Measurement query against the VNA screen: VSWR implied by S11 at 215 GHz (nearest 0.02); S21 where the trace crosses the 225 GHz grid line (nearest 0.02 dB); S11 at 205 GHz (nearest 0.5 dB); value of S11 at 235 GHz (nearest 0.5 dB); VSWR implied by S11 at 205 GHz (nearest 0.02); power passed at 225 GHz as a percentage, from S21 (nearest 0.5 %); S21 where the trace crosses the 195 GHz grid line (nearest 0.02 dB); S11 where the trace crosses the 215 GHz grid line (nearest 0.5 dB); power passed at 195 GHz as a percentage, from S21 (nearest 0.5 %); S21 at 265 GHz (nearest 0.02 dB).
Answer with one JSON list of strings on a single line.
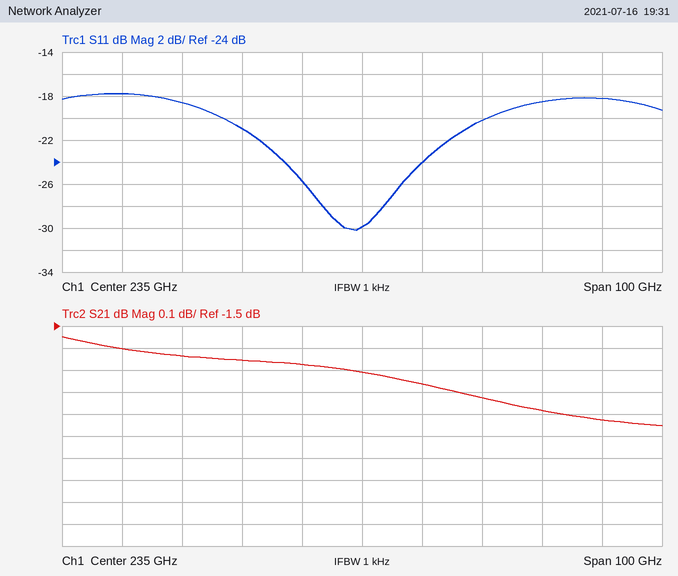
["1.20", "-1.68 dB", "-18.5 dB", "-30.0 dB", "1.26", "68.0 %", "-1.60 dB", "-21.0 dB", "69.0 %", "-1.88 dB"]
